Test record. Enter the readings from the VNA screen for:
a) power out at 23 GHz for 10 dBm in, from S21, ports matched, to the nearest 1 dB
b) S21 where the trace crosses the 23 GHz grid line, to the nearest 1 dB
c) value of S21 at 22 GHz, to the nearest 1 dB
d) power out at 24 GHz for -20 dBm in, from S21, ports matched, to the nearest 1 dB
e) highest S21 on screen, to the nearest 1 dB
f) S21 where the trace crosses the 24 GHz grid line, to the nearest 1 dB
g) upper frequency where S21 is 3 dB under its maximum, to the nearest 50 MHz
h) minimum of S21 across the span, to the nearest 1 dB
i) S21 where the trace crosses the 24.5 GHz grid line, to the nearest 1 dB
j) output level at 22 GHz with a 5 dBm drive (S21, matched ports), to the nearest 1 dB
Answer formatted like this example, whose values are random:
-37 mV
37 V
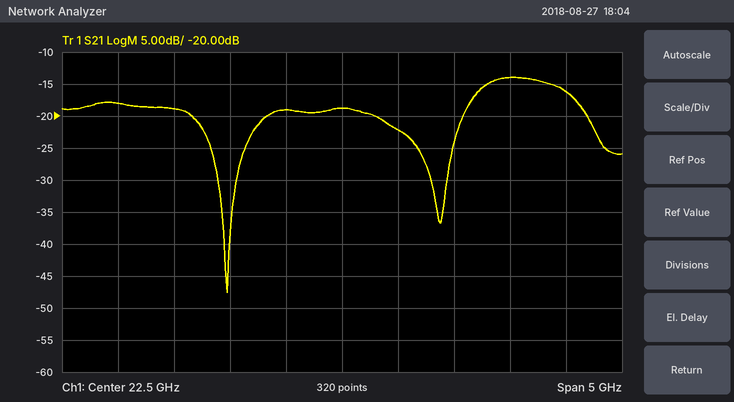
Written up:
-12 dBm
-22 dB
-19 dB
-34 dBm
-14 dB
-14 dB
24.55 GHz
-48 dB
-16 dB
-14 dBm
